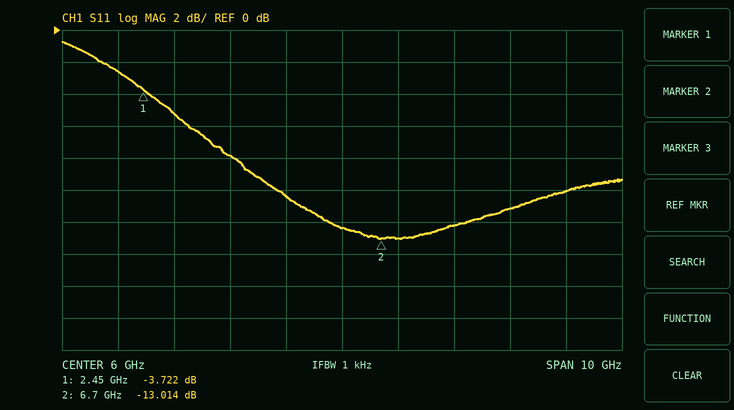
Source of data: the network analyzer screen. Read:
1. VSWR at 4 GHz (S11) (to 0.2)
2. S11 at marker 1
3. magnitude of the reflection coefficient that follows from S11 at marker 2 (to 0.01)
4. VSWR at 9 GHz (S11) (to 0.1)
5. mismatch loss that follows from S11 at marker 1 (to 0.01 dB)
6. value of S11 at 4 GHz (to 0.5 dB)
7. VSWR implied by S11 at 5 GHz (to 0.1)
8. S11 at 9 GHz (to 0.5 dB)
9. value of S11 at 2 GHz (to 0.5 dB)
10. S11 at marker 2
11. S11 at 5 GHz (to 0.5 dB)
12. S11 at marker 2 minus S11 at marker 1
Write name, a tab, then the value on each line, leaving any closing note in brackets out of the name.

VSWR at 4 GHz (S11)	2.4
S11 at marker 1	-3.722 dB
magnitude of the reflection coefficient that follows from S11 at marker 2	0.22
VSWR at 9 GHz (S11)	1.8
mismatch loss that follows from S11 at marker 1	2.40 dB
value of S11 at 4 GHz	-8.0 dB
VSWR implied by S11 at 5 GHz	1.9
S11 at 9 GHz	-11.0 dB
value of S11 at 2 GHz	-2.5 dB
S11 at marker 2	-13.014 dB
S11 at 5 GHz	-10.5 dB
S11 at marker 2 minus S11 at marker 1	-9.292 dB
